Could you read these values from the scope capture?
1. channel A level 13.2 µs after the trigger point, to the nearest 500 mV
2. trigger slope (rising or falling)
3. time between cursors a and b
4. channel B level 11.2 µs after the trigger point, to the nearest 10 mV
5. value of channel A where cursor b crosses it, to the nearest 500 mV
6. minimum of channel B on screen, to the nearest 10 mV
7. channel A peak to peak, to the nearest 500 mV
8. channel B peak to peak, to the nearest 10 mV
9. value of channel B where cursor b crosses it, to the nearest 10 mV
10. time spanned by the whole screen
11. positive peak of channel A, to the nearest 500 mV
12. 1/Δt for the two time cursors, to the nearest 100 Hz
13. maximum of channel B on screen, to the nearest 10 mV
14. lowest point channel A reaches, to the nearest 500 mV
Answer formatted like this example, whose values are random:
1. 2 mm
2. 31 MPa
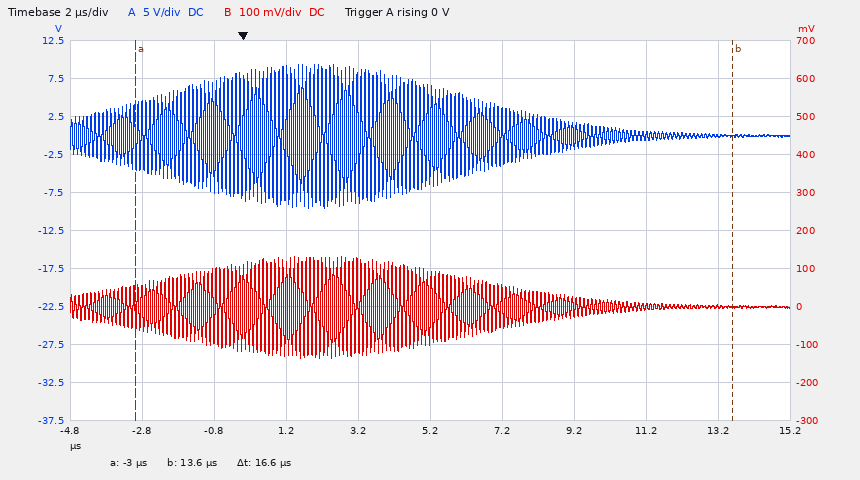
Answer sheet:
1. 0.0 V
2. rising
3. 16.6 µs
4. 0 mV
5. 0.0 V
6. -140 mV
7. 19.0 V
8. 270 mV
9. 0 mV
10. 20 µs
11. 9.5 V
12. 60.2 kHz
13. 130 mV
14. -9.5 V
